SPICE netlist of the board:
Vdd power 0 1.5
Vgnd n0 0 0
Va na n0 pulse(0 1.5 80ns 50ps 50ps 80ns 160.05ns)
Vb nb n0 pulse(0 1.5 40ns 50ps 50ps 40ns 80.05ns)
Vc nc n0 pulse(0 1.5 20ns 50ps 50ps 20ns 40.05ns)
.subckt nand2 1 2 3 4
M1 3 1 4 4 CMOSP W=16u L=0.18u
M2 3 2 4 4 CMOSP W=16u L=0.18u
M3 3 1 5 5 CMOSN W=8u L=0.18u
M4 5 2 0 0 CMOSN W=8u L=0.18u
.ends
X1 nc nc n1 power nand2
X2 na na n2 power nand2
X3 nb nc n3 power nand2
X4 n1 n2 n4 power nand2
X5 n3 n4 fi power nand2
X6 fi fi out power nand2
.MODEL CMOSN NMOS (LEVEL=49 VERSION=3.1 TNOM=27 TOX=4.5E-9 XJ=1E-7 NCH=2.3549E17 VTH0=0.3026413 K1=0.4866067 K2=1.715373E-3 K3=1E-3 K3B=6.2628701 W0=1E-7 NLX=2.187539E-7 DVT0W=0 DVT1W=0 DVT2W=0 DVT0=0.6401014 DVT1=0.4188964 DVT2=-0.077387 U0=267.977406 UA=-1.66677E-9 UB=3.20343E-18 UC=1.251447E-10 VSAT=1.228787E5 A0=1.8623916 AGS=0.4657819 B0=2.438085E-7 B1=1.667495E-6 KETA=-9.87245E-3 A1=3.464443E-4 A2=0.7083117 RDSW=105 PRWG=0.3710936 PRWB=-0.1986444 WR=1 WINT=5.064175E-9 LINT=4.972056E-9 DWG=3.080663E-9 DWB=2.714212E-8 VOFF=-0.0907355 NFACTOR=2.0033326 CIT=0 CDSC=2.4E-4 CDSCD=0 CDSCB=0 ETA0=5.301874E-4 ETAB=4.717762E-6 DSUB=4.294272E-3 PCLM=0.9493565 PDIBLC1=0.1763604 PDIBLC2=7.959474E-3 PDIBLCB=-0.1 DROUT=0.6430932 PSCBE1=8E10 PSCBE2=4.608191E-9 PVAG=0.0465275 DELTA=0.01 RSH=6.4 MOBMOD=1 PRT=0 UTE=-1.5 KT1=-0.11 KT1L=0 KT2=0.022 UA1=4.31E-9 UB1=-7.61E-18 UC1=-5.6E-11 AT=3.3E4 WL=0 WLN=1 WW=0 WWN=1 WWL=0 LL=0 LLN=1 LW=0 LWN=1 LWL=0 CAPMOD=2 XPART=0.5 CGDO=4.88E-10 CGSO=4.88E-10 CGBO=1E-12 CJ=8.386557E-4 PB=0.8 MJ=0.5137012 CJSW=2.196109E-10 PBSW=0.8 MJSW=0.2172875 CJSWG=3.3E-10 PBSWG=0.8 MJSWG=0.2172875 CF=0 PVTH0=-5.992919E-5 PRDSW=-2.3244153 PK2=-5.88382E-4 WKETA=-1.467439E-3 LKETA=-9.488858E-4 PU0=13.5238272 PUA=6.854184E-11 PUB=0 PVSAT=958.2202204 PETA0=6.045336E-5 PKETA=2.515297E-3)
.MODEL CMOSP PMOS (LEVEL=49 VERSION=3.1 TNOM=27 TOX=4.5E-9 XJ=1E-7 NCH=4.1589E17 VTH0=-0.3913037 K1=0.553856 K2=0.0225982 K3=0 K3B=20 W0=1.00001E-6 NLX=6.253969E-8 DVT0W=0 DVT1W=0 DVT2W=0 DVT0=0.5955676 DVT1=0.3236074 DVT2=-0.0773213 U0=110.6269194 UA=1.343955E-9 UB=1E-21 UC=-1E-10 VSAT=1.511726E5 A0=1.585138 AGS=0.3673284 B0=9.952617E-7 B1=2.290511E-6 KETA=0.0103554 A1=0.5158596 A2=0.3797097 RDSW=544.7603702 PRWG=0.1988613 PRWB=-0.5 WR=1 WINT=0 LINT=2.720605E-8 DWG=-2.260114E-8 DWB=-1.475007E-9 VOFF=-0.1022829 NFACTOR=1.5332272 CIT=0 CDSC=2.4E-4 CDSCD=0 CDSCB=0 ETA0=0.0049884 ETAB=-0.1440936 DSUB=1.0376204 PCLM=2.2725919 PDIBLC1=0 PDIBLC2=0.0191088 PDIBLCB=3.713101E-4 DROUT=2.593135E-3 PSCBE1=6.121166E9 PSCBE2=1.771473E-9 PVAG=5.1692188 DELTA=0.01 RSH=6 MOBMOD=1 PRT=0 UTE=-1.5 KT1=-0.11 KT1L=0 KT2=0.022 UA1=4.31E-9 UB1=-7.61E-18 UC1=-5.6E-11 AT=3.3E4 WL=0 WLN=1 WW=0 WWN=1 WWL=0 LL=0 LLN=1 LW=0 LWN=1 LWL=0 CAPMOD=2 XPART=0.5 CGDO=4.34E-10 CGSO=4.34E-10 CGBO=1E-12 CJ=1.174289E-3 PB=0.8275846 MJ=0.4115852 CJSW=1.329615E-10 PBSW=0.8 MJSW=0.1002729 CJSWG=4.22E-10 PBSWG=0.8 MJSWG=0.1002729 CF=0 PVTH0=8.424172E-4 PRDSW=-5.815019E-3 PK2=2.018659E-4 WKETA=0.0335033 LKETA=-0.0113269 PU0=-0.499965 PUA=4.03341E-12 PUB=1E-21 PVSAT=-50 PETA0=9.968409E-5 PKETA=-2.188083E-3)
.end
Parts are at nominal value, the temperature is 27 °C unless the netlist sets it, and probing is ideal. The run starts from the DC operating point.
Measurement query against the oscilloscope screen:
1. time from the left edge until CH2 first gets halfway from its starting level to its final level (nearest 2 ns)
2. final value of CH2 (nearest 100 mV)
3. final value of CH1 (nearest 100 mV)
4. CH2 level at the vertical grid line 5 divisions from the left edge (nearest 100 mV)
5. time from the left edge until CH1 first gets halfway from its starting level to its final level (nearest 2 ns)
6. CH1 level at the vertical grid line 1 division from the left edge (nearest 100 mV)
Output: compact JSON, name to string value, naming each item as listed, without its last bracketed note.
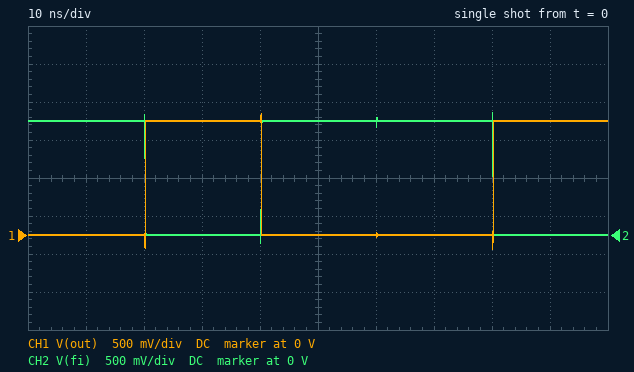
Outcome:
{"time from the left edge until CH2 first gets halfway from its starting level to its final level": "20 ns", "final value of CH2": "0 V", "final value of CH1": "1.5 V", "CH2 level at the vertical grid line 5 divisions from the left edge": "1.5 V", "time from the left edge until CH1 first gets halfway from its starting level to its final level": "20 ns", "CH1 level at the vertical grid line 1 division from the left edge": "0 V"}
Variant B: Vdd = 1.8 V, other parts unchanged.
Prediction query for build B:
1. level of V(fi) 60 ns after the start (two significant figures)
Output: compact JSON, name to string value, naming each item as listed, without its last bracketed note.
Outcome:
{"level of V(fi) 60 ns after the start": "1.8 V"}
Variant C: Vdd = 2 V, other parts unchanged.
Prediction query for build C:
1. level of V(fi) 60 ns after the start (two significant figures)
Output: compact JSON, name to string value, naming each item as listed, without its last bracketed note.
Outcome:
{"level of V(fi) 60 ns after the start": "2.0 V"}
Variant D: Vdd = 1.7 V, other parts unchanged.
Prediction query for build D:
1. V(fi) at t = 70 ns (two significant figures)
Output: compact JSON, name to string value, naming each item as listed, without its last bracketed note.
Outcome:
{"V(fi) at t = 70 ns": "1.7 V"}
